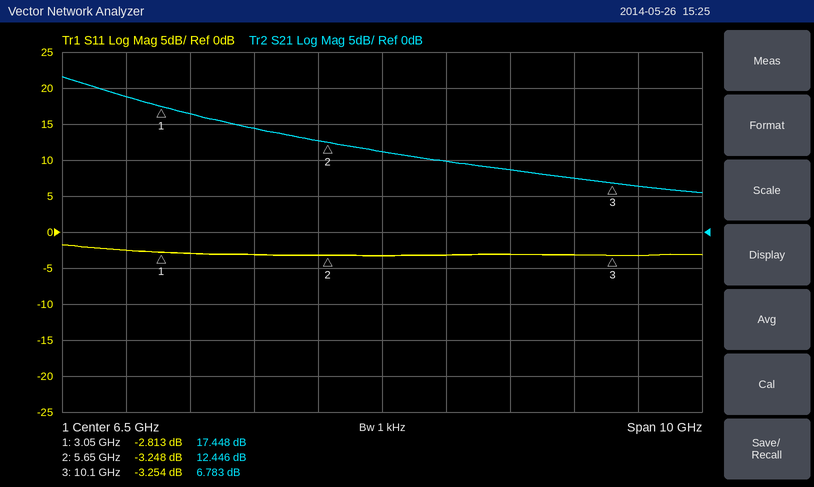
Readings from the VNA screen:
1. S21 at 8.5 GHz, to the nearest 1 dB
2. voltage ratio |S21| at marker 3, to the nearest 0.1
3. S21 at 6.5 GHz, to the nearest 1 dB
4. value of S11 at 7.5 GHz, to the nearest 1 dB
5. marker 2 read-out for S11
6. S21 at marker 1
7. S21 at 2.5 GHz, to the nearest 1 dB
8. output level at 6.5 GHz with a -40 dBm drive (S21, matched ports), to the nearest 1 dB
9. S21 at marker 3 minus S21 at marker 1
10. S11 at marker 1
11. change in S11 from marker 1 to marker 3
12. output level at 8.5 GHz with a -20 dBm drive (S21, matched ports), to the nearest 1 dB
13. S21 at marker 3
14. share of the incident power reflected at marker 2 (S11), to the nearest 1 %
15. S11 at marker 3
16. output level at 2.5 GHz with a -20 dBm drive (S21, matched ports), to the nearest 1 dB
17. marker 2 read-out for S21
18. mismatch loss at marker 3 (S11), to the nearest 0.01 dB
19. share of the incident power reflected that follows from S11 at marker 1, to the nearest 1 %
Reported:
9 dB
2.2
11 dB
-3 dB
-3.248 dB
17.448 dB
19 dB
-29 dBm
-10.665 dB
-2.813 dB
-0.441 dB
-11 dBm
6.783 dB
47 %
-3.254 dB
-1 dBm
12.446 dB
2.78 dB
52 %
